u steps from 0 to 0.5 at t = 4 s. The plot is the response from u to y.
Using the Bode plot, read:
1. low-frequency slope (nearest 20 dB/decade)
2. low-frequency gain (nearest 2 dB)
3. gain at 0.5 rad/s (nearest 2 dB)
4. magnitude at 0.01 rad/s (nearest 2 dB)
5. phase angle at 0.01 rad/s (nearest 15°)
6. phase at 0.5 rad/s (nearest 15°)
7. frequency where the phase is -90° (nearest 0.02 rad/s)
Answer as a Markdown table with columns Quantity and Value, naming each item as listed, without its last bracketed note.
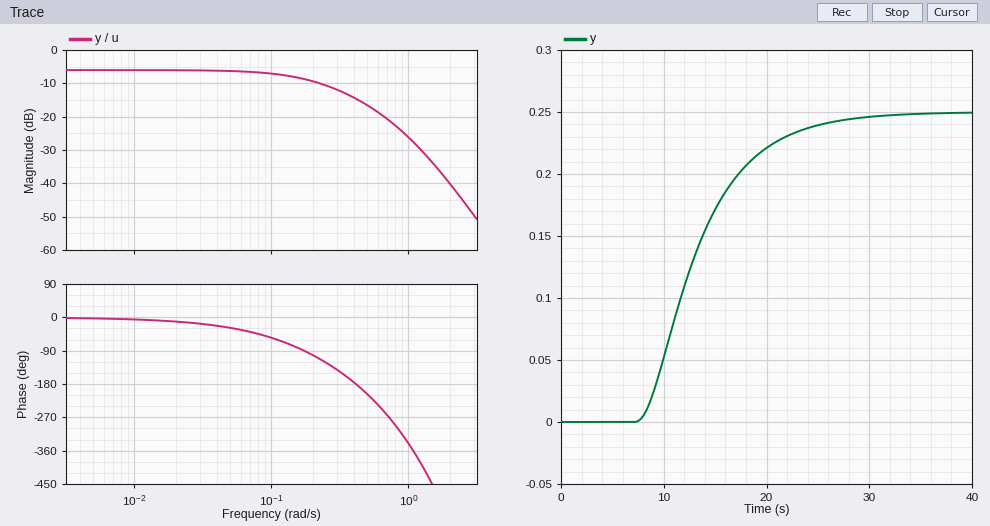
| Quantity | Value |
|---|---|
| low-frequency slope | 0 dB/decade |
| low-frequency gain | -6 dB |
| gain at 0.5 rad/s | -16 dB |
| magnitude at 0.01 rad/s | -6 dB |
| phase angle at 0.01 rad/s | 0° |
| phase at 0.5 rad/s | -210° |
| frequency where the phase is -90° | 0.18 rad/s |
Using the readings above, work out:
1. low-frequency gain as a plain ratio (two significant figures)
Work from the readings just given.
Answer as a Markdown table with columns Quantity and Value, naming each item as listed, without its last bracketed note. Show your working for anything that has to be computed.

| Quantity | Value |
|---|---|
| low-frequency gain as a plain ratio | 10^(-6 / 20) = 0.50 |
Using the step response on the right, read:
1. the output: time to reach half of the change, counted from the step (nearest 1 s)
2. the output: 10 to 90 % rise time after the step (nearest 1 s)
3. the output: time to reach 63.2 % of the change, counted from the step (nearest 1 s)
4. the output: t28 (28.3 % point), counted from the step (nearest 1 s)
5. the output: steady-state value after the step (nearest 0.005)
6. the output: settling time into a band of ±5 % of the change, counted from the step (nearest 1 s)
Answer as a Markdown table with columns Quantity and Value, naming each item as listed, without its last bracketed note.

| Quantity | Value |
|---|---|
| the output: time to reach half of the change, counted from the step | 9 s |
| the output: 10 to 90 % rise time after the step | 12 s |
| the output: time to reach 63.2 % of the change, counted from the step | 10 s |
| the output: t28 (28.3 % point), counted from the step | 7 s |
| the output: steady-state value after the step | 0.250 |
| the output: settling time into a band of ±5 % of the change, counted from the step | 20 s |
